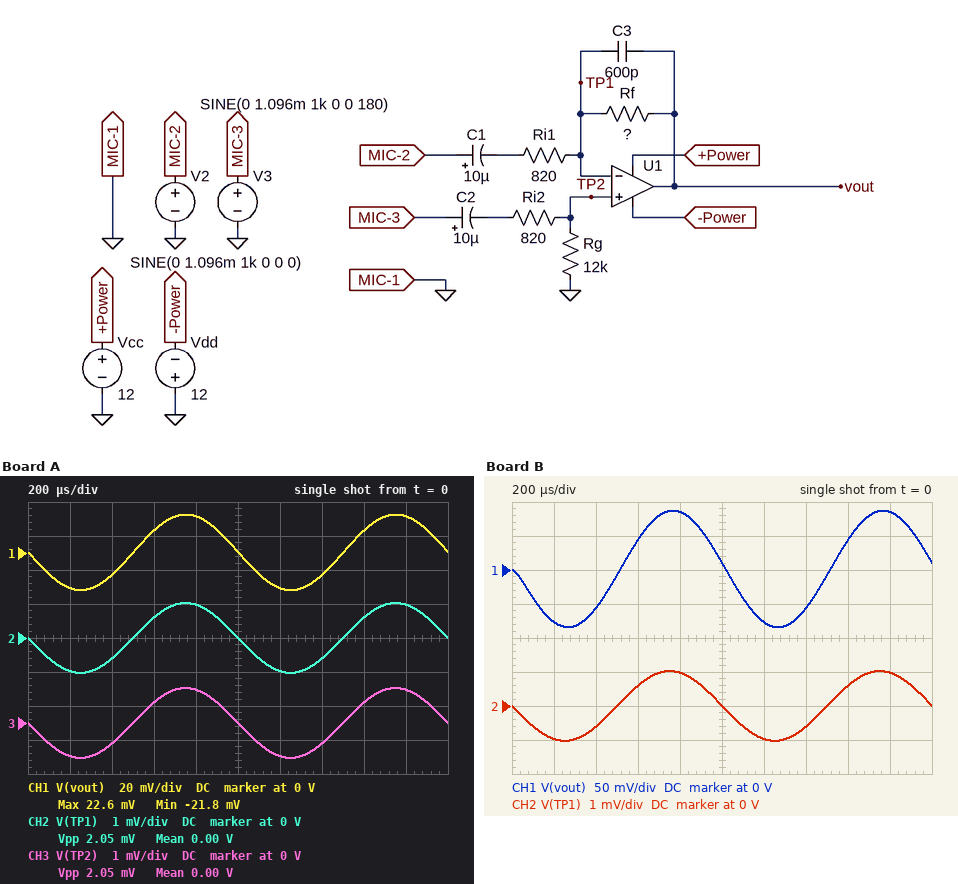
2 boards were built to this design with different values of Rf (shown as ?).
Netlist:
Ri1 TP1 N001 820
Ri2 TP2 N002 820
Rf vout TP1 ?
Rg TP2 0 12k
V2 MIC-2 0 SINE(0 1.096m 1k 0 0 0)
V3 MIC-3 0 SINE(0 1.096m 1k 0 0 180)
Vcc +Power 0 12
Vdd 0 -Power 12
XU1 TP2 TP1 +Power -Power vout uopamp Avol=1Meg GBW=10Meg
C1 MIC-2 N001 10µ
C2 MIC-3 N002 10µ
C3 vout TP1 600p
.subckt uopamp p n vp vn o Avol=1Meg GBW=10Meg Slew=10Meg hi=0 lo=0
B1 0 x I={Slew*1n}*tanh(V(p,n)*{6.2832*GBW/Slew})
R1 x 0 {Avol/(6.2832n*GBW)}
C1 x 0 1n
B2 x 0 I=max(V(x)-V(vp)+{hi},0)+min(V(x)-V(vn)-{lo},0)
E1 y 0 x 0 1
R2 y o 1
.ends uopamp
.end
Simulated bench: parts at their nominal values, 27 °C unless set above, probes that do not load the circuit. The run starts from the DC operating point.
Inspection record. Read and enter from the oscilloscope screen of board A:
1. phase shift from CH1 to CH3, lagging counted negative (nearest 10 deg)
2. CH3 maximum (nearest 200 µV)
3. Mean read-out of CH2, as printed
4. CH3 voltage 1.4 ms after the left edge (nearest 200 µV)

0 deg
1.0 mV
0.00 V
-600 µV
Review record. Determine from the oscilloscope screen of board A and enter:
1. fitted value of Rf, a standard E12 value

8.2 kΩ
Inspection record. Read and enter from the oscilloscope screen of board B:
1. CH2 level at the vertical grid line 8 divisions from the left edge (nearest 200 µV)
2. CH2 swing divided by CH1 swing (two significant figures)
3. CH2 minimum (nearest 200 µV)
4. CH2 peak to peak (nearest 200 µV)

600 µV
0.012
-1.0 mV
2.0 mV
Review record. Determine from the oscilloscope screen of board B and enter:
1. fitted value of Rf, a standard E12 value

33 kΩ
